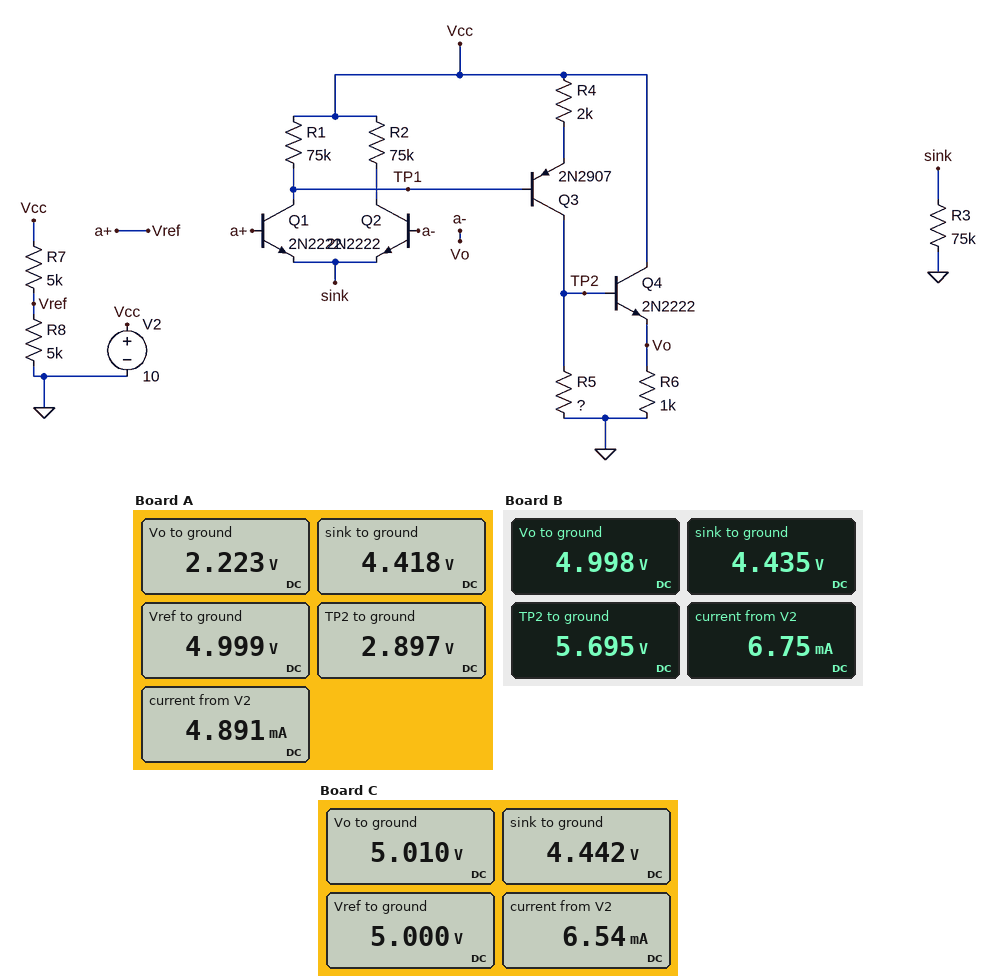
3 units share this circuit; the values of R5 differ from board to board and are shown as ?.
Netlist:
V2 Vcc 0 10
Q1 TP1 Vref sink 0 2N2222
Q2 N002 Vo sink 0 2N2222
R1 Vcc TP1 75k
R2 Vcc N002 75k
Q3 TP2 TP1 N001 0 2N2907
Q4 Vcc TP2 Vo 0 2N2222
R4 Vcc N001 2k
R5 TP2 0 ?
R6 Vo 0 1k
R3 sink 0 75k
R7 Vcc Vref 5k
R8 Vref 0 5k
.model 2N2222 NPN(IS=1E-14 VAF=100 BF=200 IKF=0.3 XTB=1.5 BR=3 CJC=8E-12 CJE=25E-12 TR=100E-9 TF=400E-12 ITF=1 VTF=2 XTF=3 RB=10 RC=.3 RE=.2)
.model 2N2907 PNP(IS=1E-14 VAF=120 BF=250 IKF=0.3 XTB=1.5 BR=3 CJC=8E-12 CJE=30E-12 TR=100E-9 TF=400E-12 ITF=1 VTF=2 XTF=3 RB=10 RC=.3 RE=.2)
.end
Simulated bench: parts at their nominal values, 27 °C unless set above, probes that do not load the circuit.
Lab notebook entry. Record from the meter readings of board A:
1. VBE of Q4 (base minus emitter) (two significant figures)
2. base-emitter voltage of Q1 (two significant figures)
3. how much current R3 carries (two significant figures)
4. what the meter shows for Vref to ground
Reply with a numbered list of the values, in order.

1. 670 mV
2. 580 mV
3. 59 µA
4. 4.999 V
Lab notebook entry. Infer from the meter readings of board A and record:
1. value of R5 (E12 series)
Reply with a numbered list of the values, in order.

1. 1.8 kΩ
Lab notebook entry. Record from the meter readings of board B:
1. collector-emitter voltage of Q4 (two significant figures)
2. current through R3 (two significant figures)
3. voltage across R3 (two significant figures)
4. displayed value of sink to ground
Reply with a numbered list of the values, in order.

1. 5.0 V
2. 59 µA
3. 4.4 V
4. 4.435 V
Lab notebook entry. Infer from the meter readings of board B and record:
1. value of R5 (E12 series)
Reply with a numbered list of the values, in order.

1. 8.2 kΩ
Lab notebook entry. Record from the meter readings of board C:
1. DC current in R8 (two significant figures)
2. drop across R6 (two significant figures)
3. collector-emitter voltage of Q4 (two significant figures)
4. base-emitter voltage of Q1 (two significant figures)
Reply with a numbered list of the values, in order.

1. 1.0 mA
2. 5.0 V
3. 5.0 V
4. 560 mV
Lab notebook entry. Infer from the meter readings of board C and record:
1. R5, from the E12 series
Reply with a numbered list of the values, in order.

1. 12 kΩ
